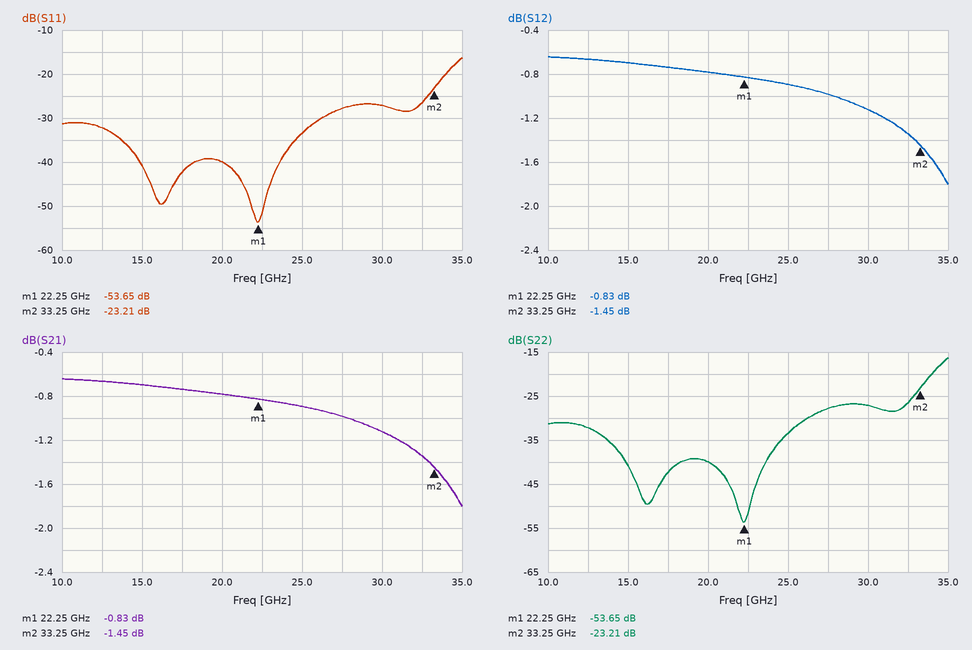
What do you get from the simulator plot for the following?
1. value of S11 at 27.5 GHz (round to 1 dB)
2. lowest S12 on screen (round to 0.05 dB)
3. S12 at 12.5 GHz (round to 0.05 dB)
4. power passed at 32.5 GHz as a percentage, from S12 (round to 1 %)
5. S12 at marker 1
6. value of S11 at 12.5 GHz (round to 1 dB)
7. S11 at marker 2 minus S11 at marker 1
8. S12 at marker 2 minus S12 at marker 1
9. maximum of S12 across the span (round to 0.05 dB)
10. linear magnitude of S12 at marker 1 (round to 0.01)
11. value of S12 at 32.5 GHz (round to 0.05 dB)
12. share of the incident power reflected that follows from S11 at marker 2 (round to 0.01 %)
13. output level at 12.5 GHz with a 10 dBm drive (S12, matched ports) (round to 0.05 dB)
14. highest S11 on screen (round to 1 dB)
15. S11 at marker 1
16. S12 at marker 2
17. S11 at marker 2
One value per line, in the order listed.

-28 dB
-1.80 dB
-0.65 dB
73 %
-0.83 dB
-32 dB
30.44 dB
-0.62 dB
-0.65 dB
0.91
-1.35 dB
0.48 %
9.35 dBm
-16 dB
-53.65 dB
-1.45 dB
-23.21 dB
